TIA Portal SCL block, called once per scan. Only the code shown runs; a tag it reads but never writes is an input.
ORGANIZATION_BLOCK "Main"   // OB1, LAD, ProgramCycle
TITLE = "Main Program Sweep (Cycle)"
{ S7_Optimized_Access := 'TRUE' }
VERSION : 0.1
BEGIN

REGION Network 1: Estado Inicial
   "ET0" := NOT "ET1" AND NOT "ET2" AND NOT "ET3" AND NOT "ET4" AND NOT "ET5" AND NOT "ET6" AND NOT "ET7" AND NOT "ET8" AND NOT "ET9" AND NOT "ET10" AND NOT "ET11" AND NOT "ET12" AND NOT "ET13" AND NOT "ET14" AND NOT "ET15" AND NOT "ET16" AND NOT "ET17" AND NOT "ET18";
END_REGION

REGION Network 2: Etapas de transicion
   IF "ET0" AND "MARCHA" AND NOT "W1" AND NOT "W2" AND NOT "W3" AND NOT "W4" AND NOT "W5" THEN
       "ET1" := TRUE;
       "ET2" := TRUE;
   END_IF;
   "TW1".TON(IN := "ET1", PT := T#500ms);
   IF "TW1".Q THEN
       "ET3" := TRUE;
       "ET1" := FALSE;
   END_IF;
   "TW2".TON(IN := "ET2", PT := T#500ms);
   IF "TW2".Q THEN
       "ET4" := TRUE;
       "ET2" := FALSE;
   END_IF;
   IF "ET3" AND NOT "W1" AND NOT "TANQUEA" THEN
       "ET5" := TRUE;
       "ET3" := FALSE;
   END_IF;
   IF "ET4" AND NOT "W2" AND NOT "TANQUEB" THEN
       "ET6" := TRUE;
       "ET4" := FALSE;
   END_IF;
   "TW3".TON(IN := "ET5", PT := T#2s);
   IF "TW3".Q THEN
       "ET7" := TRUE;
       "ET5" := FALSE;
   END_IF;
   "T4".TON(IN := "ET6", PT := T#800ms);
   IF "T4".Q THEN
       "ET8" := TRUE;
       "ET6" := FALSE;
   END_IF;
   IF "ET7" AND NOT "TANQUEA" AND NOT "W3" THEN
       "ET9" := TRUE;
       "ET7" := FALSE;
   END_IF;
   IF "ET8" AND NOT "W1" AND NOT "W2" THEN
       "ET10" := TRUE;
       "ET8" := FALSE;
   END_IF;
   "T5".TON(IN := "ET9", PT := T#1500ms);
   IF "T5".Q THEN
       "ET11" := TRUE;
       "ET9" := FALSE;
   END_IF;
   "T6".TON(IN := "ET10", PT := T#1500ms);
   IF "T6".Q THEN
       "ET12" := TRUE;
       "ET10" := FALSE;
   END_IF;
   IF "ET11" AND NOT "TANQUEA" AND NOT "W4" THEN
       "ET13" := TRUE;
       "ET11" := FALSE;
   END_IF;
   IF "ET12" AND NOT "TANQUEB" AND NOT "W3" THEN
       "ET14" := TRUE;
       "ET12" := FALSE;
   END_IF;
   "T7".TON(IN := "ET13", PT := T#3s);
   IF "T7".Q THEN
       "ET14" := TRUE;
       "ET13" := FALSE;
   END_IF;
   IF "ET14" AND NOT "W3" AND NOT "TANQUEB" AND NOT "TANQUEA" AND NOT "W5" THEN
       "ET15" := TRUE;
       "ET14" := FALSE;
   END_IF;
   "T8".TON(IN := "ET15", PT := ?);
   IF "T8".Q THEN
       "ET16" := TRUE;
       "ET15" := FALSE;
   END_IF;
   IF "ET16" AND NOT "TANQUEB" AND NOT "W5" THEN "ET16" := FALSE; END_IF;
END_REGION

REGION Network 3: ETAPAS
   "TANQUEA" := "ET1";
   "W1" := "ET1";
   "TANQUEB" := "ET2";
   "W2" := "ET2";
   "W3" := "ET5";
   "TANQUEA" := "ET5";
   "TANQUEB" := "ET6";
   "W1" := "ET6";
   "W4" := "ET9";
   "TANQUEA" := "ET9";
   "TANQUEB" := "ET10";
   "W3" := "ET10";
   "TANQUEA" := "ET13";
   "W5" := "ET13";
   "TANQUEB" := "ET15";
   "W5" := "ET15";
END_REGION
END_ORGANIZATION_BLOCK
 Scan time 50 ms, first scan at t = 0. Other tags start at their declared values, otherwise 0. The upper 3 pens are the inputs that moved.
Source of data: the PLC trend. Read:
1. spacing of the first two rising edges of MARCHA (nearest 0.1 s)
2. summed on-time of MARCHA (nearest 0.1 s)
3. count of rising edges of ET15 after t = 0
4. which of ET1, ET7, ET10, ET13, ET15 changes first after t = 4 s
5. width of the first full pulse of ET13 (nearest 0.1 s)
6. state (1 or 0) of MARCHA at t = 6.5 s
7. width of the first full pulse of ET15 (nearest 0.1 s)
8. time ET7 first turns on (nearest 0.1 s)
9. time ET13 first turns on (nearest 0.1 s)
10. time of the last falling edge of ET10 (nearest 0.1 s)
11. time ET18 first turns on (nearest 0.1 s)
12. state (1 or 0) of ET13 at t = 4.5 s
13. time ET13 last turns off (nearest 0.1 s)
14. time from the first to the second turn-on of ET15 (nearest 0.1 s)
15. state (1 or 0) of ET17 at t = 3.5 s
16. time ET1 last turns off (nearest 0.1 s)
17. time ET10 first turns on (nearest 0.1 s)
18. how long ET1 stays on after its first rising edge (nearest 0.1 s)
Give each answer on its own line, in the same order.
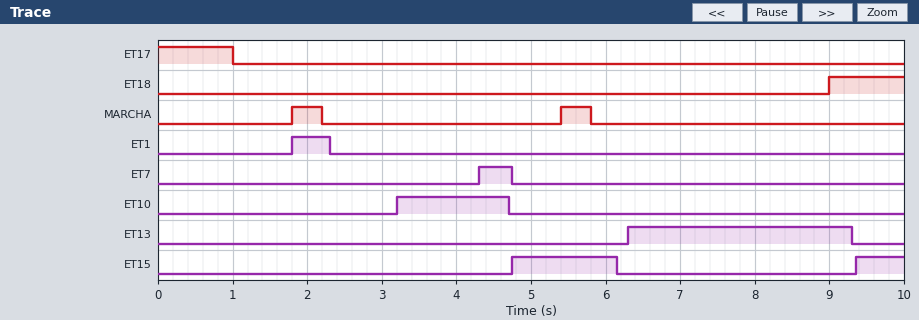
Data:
3.6 s
0.8 s
2
ET7
3.0 s
0
1.4 s
4.3 s
6.3 s
4.7 s
9.0 s
0
9.3 s
4.6 s
0
2.3 s
3.2 s
0.5 s
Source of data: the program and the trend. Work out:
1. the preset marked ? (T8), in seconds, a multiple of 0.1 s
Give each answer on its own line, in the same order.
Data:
1.4 s
